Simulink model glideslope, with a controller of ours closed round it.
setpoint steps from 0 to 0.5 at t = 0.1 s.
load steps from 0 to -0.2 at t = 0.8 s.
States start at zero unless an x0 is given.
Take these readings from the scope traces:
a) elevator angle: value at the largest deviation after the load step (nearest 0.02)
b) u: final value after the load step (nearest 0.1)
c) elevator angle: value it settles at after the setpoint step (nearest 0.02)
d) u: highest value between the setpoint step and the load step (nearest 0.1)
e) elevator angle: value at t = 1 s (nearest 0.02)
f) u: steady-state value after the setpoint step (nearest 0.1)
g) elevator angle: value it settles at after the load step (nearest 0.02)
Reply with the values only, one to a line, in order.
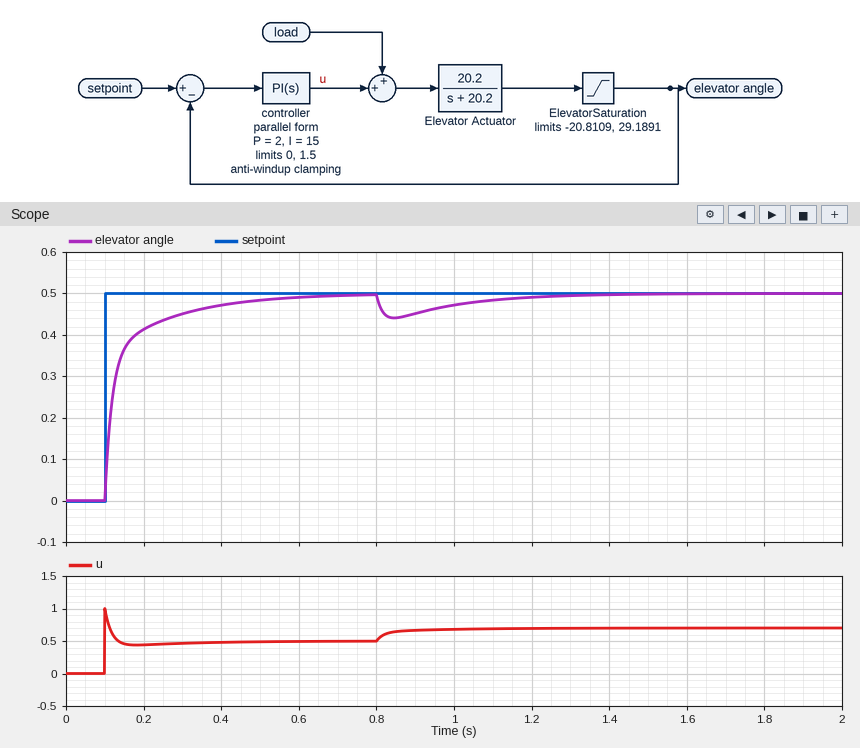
0.44
0.7
0.50
1.0
0.48
0.5
0.50
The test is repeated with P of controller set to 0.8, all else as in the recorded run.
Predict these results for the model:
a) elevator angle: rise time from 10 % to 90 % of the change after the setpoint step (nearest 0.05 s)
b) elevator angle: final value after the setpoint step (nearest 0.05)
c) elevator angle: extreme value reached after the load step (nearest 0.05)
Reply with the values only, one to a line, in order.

0.15 s
0.50
0.40
